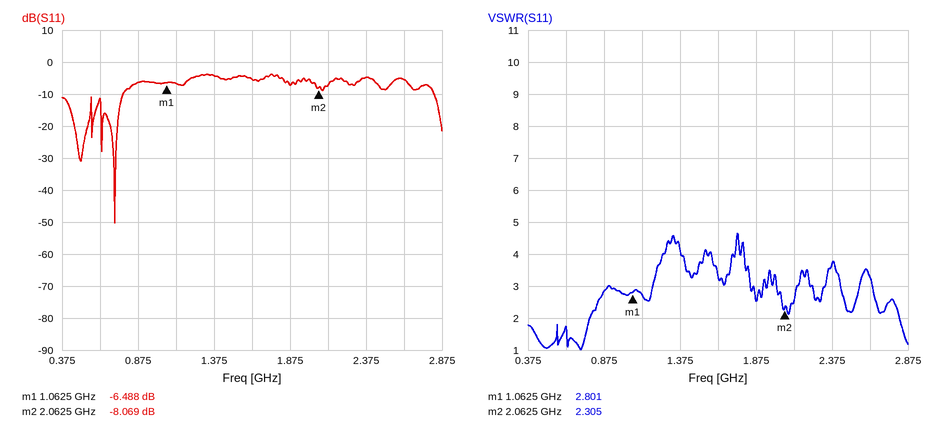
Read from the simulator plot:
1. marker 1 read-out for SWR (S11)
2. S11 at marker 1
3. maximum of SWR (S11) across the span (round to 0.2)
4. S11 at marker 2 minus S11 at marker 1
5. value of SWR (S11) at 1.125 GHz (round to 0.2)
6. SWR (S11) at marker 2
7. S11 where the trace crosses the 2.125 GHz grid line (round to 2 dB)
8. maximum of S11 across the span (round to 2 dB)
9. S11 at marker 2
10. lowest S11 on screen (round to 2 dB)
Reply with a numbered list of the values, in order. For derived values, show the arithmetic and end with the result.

1. 2.801
2. -6.488 dB
3. 4.6
4. -8.069 − (-6.488) = -1.581 dB
5. 2.8
6. 2.305
7. -8 dB
8. -4 dB
9. -8.069 dB
10. -50 dB
